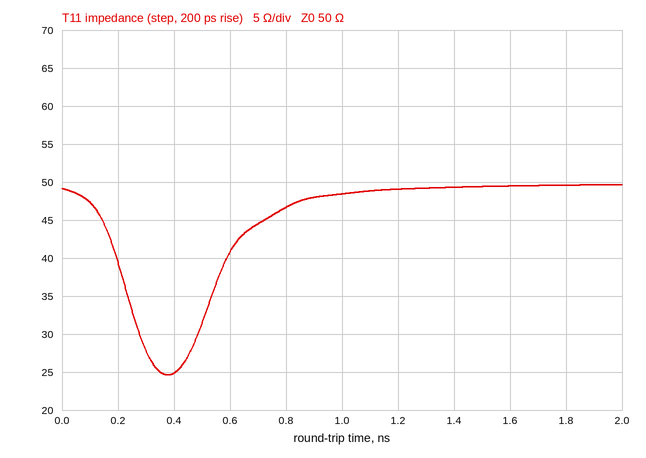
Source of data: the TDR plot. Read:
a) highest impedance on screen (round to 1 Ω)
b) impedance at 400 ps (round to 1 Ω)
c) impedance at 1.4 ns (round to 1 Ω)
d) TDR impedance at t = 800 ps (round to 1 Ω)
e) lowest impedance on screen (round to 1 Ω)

50 Ω
25 Ω
49 Ω
47 Ω
25 Ω
